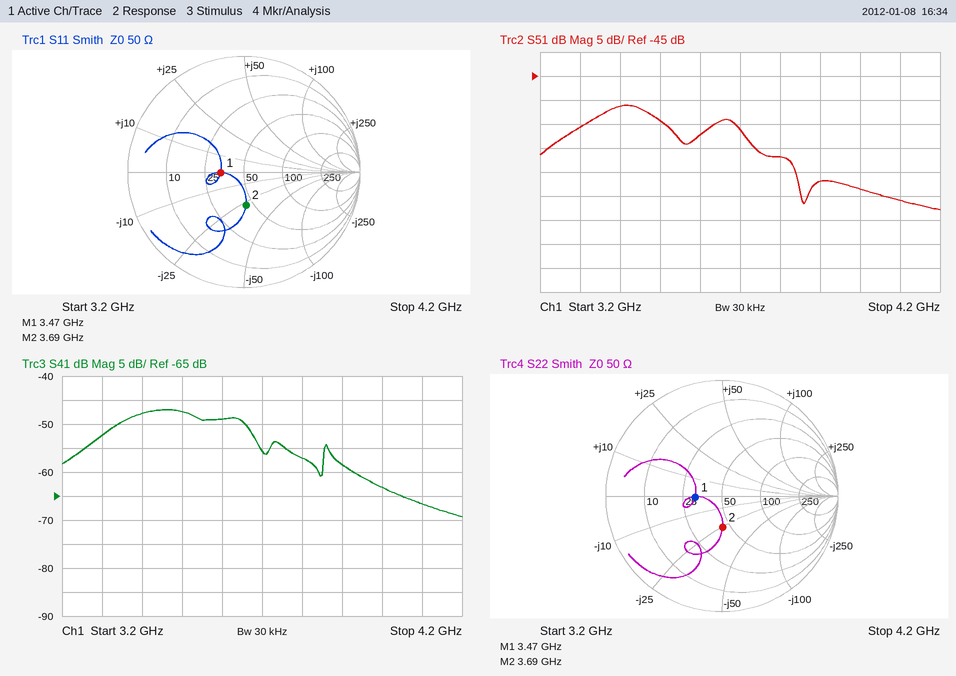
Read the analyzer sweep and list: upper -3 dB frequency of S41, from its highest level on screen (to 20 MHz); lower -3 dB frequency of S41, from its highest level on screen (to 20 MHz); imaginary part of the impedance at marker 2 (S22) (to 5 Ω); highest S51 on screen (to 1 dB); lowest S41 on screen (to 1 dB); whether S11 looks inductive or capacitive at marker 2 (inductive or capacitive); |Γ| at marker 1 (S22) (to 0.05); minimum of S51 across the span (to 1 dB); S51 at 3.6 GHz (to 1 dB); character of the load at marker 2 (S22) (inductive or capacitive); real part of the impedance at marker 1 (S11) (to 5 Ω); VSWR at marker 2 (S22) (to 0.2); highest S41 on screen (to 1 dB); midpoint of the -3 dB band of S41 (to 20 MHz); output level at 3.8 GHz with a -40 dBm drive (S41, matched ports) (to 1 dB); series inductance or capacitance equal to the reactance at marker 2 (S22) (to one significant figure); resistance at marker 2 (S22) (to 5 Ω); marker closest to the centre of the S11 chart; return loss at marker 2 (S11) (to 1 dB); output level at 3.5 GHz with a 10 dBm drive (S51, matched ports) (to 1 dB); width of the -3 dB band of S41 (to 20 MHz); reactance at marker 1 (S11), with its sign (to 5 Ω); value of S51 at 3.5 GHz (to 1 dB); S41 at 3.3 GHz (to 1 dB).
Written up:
3.66 GHz
3.34 GHz
-25 Ω
-51 dB
-69 dB
capacitive
0.25
-73 dB
-57 dB
capacitive
35 Ω
1.8
-47 dB
3.50 GHz
-97 dBm
2 pF
45 Ω
marker 1
11 dB
-44 dBm
320 MHz
0 Ω
-54 dB
-52 dB
